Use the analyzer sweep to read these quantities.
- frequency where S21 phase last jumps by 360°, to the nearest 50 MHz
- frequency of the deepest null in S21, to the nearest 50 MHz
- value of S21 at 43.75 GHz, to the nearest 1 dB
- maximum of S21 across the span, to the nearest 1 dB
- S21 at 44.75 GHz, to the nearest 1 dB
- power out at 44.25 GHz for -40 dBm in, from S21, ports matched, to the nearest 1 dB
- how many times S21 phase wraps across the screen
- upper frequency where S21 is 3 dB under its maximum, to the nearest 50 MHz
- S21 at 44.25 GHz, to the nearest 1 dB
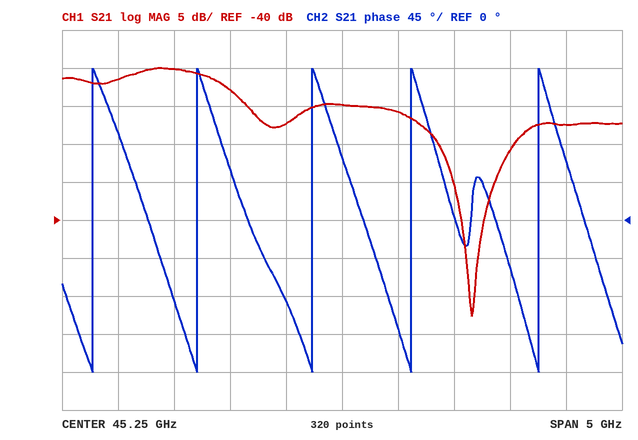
47.00 GHz
46.40 GHz
-20 dB
-20 dB
-27 dB
-63 dBm
5
44.25 GHz
-23 dB
